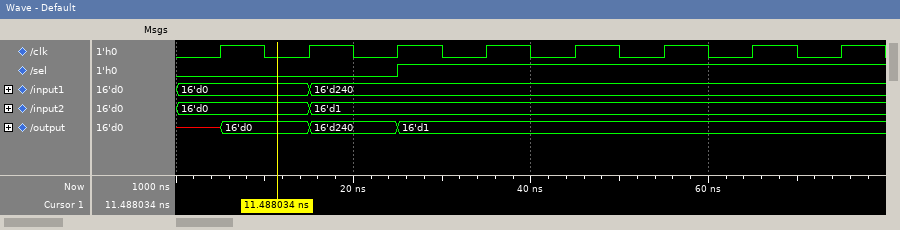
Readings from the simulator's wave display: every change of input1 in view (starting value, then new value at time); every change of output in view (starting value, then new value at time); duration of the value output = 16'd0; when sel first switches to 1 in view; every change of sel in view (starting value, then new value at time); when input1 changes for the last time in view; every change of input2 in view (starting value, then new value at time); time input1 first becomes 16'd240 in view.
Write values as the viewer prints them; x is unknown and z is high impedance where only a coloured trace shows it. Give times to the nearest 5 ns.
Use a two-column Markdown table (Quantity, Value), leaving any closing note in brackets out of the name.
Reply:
| Quantity | Value |
|---|---|
| every change of input1 in view | 16'd0, 16'd240 at 15 ns |
| every change of output in view | x, 16'd0 at 5 ns, 16'd240 at 15 ns, 16'd1 at 25 ns |
| duration of the value output = 16'd0 | 10 ns |
| when sel first switches to 1 in view | 25 ns |
| every change of sel in view | 0, 1 at 25 ns |
| when input1 changes for the last time in view | 15 ns |
| every change of input2 in view | 16'd0, 16'd1 at 15 ns |
| time input1 first becomes 16'd240 in view | 15 ns |
